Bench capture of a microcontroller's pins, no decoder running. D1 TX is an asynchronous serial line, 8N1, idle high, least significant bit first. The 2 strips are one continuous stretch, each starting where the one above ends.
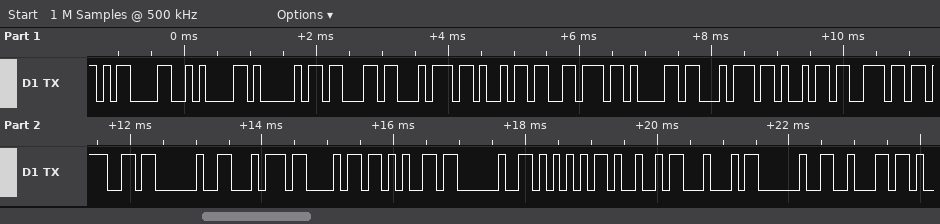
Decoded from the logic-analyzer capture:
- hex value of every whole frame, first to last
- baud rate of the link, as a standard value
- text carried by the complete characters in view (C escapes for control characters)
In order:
0x0D 0x0A 0x41 0x63 0x74 0x69 0x76 0x61 0x74 0x69 0x6E 0x67 0x20 0x74 0x68 0x65 0x20 0x55 0x49 0x44 0x20 0x62
9600 baud
"\r\nActivating the UID b"
